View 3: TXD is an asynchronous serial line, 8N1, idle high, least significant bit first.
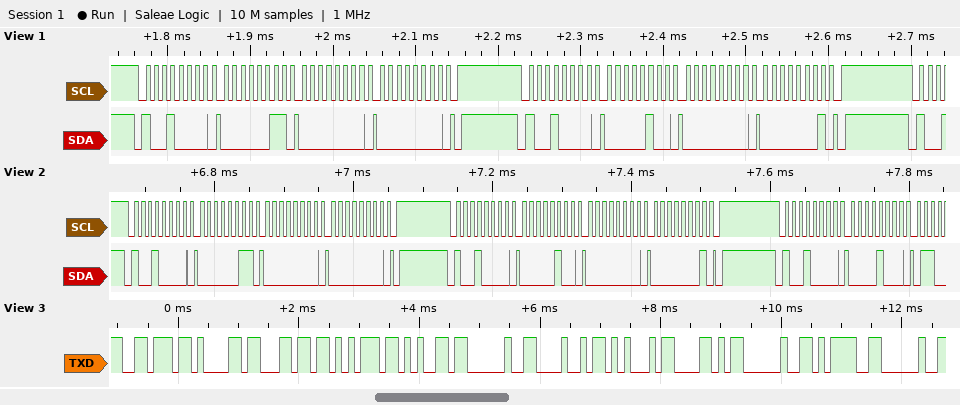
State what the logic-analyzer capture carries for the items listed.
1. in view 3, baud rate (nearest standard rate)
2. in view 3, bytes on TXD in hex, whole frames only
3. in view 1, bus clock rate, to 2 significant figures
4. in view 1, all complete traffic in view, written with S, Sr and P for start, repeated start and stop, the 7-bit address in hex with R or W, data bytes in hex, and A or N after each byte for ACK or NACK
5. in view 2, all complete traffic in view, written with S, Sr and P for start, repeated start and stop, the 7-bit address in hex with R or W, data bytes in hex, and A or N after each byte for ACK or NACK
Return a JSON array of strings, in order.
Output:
["9600 baud", "76 61 6C 75 65 20 48 45 58 20 3D 20", "100 kHz", "S 48W A 03 A 00 A 00 A P S 48W A 04 A 00 A 01 A P", "S 48W A 03 A 00 A 00 A P S 48W A 04 A 00 A 01 A P S 48W A 08 A"]
